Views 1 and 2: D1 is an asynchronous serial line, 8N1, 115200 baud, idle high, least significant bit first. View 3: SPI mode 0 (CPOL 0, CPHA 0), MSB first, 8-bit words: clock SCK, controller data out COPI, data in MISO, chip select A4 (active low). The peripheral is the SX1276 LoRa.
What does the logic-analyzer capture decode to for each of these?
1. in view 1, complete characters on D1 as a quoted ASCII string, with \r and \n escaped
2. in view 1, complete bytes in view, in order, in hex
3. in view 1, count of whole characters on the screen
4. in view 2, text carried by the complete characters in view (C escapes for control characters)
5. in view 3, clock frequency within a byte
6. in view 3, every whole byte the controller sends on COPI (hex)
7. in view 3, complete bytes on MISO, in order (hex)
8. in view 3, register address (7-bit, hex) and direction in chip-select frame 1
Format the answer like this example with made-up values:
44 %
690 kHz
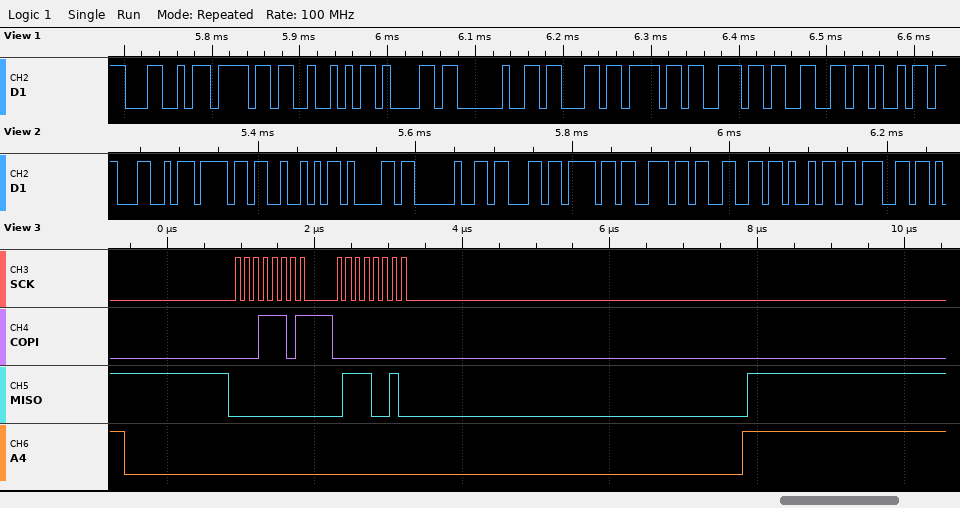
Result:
"LoRa confi"
0x4C 0x6F 0x52 0x61 0x20 0x63 0x6F 0x6E 0x66 0x69
10
"LoRa config"
8 MHz
0x1D 0x00
0x00 0x72
0x1D read
